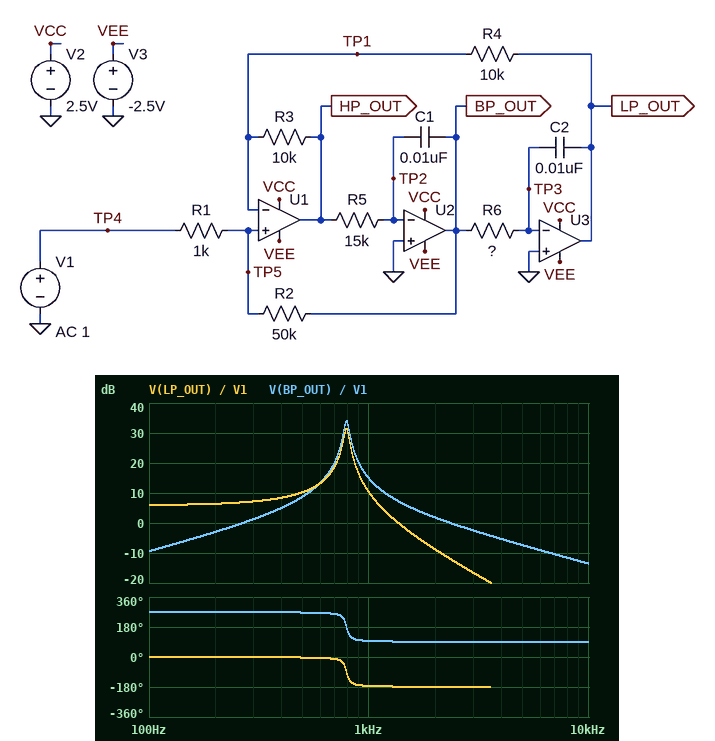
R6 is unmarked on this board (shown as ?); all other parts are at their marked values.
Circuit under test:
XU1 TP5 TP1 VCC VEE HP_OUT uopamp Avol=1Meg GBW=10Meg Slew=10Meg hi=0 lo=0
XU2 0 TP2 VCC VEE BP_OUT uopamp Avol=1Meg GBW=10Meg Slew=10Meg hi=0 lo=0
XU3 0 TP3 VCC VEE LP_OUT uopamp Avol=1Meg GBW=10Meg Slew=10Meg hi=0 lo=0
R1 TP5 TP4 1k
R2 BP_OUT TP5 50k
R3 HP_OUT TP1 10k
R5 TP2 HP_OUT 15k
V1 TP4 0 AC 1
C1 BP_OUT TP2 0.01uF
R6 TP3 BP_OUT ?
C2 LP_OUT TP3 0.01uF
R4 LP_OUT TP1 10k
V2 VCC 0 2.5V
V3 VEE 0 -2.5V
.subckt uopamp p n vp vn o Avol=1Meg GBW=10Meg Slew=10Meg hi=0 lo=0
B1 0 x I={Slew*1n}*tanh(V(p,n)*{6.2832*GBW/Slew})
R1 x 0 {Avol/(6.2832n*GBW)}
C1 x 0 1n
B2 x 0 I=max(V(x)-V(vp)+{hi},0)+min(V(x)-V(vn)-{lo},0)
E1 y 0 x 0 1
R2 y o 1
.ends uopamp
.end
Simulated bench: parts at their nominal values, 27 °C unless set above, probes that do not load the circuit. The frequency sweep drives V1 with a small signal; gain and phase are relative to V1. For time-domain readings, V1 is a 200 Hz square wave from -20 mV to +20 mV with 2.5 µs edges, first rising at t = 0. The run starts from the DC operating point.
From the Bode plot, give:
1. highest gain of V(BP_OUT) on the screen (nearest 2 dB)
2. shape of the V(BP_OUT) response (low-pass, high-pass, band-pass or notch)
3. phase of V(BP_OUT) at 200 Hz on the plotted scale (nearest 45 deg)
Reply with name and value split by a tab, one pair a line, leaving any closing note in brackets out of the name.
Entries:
highest gain of V(BP_OUT) on the screen	34 dB
shape of the V(BP_OUT) response	band-pass
phase of V(BP_OUT) at 200 Hz on the plotted scale	270 deg
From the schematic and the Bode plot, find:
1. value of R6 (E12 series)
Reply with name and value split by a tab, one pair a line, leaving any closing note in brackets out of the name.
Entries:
value of R6	27 kΩ
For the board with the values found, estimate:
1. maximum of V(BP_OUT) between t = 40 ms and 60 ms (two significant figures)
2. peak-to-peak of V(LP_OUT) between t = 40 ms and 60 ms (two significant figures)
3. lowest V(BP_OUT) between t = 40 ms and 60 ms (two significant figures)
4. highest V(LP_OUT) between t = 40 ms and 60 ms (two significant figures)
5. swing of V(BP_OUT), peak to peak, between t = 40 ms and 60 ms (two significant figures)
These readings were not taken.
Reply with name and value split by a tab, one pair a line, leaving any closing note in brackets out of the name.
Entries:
maximum of V(BP_OUT) between t = 40 ms and 60 ms	59 mV
peak-to-peak of V(LP_OUT) between t = 40 ms and 60 ms	160 mV
lowest V(BP_OUT) between t = 40 ms and 60 ms	-59 mV
highest V(LP_OUT) between t = 40 ms and 60 ms	81 mV
swing of V(BP_OUT), peak to peak, between t = 40 ms and 60 ms	120 mV
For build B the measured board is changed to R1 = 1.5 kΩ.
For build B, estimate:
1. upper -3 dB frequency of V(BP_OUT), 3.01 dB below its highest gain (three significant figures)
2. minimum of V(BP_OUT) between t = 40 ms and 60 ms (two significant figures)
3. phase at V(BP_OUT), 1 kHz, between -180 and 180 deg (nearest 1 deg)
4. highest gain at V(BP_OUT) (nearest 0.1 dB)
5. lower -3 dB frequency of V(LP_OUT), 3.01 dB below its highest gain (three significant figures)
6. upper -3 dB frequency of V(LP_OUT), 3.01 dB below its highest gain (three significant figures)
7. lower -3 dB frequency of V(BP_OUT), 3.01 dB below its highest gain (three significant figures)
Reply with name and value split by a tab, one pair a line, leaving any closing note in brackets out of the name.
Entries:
upper -3 dB frequency of V(BP_OUT), 3.01 dB below its highest gain	822 Hz
minimum of V(BP_OUT) between t = 40 ms and 60 ms	-61 mV
phase at V(BP_OUT), 1 kHz, between -180 and 180 deg	99 deg
highest gain at V(BP_OUT)	30.5 dB
lower -3 dB frequency of V(LP_OUT), 3.01 dB below its highest gain	758 Hz
upper -3 dB frequency of V(LP_OUT), 3.01 dB below its highest gain	820 Hz
lower -3 dB frequency of V(BP_OUT), 3.01 dB below its highest gain	761 Hz
